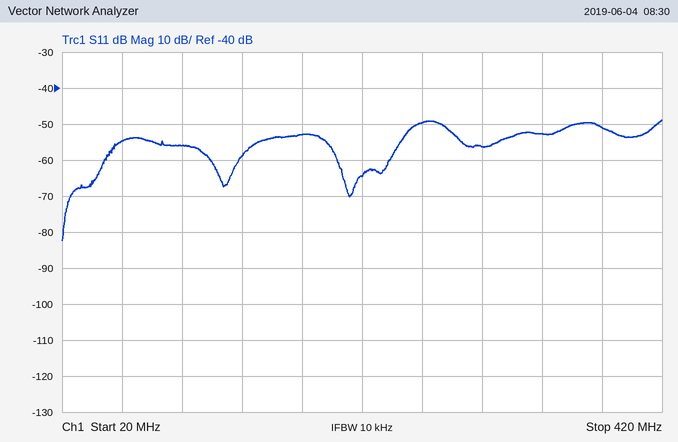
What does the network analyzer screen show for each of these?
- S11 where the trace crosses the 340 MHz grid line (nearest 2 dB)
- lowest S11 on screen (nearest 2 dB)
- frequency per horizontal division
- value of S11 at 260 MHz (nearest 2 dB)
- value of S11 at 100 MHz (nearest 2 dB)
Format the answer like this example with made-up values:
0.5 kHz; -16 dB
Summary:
-52 dB; -82 dB; 40 MHz; -50 dB; -56 dB
